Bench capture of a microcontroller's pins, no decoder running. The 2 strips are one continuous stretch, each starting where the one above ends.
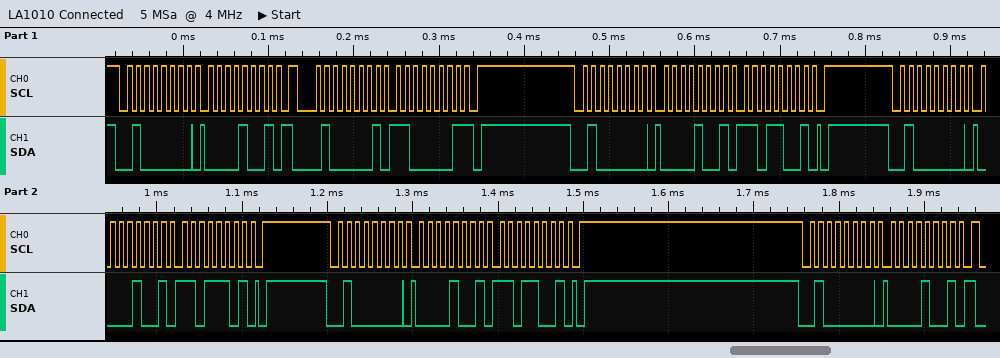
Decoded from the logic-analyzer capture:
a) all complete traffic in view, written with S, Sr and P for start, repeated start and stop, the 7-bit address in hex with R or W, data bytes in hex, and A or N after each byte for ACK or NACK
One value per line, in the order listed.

S 20W A 09 A Sr 20R A C1 N P S 20W A 09 A D9 A P S 20W A 09 A DD A P S 20W A 09 A D9 A P S 20W A 09 A
